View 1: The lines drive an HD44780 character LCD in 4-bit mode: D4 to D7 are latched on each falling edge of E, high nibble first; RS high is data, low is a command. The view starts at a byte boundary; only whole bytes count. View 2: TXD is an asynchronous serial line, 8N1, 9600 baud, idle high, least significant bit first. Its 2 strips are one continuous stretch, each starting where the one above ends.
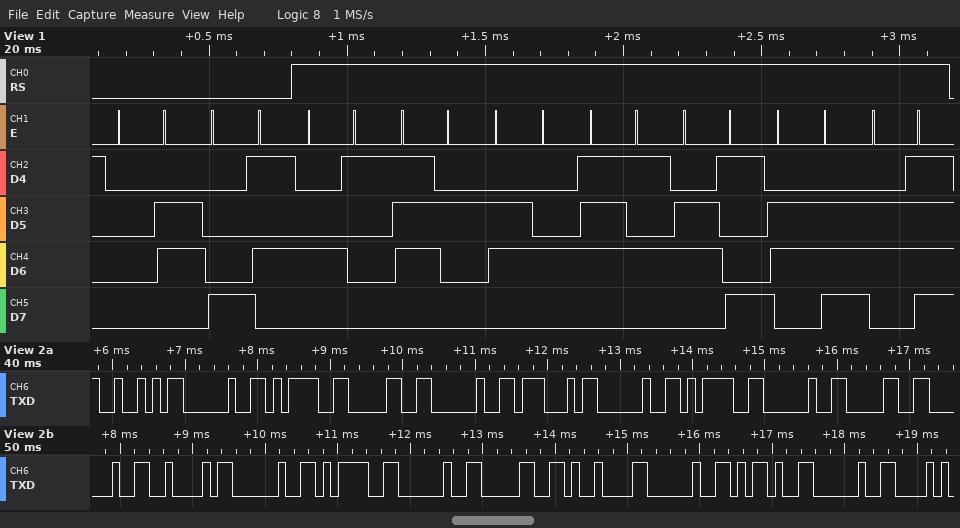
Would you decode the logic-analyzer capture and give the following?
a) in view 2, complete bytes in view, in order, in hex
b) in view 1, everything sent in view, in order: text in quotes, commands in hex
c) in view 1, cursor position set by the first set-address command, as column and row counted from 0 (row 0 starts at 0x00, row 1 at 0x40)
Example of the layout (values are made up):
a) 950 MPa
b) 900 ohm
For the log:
a) 52 20 3D 30 20 47 20 3D 20 30 20 42 20 3D 20 30 09 20 2D 20
b) 0x06 0x85 "Arduino"
c) column 5, row 0
